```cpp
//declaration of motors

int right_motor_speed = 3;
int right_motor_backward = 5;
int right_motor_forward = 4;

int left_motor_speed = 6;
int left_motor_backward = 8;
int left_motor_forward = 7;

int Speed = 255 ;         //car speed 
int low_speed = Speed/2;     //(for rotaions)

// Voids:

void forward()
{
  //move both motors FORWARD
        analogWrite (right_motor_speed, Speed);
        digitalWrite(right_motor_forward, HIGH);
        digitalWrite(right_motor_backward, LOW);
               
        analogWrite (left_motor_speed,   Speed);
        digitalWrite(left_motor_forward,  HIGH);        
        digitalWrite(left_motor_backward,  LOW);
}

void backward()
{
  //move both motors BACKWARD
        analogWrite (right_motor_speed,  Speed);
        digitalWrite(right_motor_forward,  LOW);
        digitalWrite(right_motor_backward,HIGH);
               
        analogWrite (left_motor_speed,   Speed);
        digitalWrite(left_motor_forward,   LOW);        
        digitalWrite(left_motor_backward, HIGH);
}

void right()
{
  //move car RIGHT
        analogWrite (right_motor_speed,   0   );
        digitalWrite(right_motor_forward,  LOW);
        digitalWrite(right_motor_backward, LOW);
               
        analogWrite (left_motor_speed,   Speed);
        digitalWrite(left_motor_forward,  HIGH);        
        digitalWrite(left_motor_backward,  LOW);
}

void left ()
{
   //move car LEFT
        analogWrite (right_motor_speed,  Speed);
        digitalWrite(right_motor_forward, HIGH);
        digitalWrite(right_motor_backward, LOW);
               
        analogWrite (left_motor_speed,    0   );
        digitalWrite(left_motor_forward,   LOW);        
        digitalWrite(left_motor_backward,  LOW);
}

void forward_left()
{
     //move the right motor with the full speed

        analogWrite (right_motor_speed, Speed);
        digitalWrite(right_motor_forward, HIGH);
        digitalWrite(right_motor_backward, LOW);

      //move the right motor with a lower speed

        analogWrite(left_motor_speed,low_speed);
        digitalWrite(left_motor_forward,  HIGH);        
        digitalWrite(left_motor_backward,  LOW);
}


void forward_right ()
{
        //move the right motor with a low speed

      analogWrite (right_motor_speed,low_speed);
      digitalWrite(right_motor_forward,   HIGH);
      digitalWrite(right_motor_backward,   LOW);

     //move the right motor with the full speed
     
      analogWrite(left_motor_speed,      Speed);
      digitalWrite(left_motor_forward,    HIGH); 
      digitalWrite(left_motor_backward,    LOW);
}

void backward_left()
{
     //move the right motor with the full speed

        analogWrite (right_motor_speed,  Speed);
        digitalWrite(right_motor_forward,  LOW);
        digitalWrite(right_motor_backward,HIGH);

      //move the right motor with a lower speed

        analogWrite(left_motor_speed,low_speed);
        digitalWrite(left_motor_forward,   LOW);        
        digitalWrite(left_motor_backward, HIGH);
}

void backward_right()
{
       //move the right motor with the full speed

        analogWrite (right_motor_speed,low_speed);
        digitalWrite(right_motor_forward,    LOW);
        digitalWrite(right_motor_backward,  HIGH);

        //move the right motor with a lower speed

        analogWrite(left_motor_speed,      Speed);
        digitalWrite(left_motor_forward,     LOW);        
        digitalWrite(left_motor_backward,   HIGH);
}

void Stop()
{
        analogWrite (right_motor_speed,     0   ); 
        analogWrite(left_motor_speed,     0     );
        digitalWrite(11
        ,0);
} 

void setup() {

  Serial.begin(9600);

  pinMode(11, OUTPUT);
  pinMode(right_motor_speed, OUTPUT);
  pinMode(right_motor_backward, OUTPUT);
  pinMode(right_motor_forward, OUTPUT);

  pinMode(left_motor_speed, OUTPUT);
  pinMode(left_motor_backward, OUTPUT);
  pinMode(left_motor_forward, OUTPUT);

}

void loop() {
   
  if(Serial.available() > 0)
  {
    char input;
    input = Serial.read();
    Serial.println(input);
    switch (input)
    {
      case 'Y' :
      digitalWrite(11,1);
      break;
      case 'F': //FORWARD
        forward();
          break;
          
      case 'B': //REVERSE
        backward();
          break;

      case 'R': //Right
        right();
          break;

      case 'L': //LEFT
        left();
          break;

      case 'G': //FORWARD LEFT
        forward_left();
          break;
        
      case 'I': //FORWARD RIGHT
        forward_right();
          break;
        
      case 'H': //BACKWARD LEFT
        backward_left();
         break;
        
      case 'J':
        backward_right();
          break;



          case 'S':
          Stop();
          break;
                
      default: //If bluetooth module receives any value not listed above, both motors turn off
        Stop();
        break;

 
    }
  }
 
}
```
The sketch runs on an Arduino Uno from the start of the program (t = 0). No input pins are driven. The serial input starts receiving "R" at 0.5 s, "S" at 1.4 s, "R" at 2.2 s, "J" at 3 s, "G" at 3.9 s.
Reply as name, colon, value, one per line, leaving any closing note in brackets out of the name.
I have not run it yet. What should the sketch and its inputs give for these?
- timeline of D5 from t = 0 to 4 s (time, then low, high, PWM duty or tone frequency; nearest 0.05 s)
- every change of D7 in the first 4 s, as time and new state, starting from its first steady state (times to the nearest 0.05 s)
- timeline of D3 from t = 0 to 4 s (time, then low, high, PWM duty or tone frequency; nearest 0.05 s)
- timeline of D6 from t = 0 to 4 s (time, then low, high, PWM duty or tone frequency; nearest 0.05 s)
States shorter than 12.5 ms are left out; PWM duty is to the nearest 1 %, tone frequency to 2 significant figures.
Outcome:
timeline of D5 from t = 0 to 4 s: 0 s low; 3 s high; 3.9 s low
every change of D7 in the first 4 s, as time and new state, starting from its first steady state: 0 s low; 0.5 s high; 3 s low; 3.9 s high
timeline of D3 from t = 0 to 4 s: 0 s low; 3 s PWM 50 %; 3.9 s high
timeline of D6 from t = 0 to 4 s: 0 s low; 0.5 s high; 1.4 s low; 2.2 s high; 3.9 s PWM 50 %
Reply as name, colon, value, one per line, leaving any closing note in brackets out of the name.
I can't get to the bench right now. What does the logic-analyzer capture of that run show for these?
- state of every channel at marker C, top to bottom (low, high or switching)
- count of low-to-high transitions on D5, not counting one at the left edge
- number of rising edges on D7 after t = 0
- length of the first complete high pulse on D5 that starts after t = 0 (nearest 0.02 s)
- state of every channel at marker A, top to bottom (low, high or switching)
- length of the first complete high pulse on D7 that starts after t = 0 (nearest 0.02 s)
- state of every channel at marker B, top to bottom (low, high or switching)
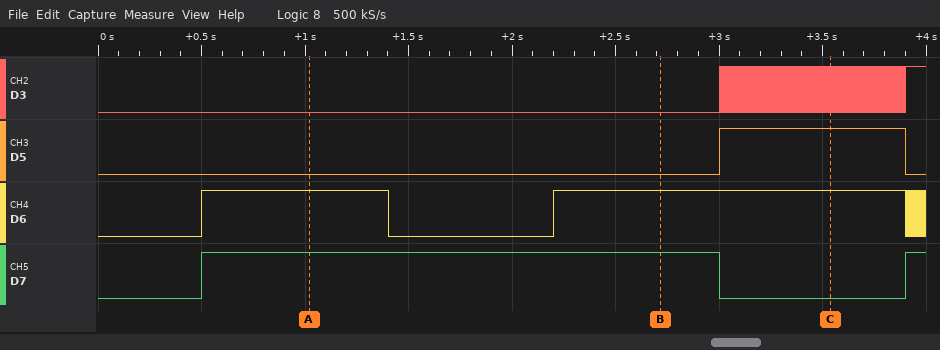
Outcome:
state of every channel at marker C, top to bottom: D3 switching, D5 high, D6 high, D7 low
count of low-to-high transitions on D5, not counting one at the left edge: 1
number of rising edges on D7 after t = 0: 2
length of the first complete high pulse on D5 that starts after t = 0: 0.90 s
state of every channel at marker A, top to bottom: D3 low, D5 low, D6 high, D7 high
length of the first complete high pulse on D7 that starts after t = 0: 2.50 s
state of every channel at marker B, top to bottom: D3 low, D5 low, D6 high, D7 high
